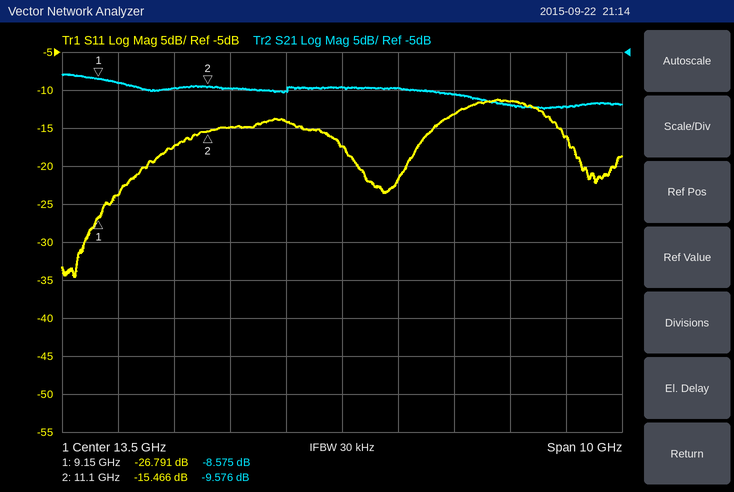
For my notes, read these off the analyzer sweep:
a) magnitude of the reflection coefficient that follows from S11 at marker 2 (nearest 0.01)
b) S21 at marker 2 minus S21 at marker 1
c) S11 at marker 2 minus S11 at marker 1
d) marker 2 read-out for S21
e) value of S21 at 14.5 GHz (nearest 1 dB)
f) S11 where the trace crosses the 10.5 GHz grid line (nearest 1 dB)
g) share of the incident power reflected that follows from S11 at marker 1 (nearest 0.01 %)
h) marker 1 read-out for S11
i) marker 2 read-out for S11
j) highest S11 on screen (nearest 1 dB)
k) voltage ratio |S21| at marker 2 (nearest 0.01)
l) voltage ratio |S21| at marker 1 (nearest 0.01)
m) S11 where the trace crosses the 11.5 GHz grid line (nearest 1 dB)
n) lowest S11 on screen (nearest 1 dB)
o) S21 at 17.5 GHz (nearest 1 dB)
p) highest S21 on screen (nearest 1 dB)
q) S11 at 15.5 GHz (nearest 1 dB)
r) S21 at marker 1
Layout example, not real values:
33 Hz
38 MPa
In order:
0.17
-1.001 dB
11.325 dB
-9.576 dB
-10 dB
-17 dB
0.21 %
-26.791 dB
-15.466 dB
-11 dB
0.33
0.37
-15 dB
-35 dB
-12 dB
-8 dB
-13 dB
-8.575 dB
